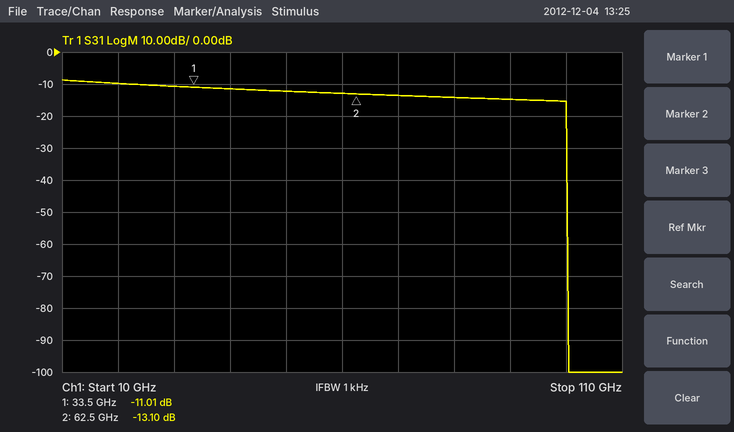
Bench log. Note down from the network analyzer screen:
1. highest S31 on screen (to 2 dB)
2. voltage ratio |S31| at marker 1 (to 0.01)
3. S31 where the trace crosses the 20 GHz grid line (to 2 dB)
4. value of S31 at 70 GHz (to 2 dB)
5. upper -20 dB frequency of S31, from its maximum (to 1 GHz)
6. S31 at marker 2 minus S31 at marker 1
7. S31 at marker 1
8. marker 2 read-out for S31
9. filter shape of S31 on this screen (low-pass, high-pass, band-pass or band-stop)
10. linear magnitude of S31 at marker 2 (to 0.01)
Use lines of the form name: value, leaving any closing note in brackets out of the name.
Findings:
highest S31 on screen: -8 dB
voltage ratio |S31| at marker 1: 0.28
S31 where the trace crosses the 20 GHz grid line: -10 dB
value of S31 at 70 GHz: -14 dB
upper -20 dB frequency of S31, from its maximum: 100 GHz
S31 at marker 2 minus S31 at marker 1: -2.09 dB
S31 at marker 1: -11.01 dB
marker 2 read-out for S31: -13.10 dB
filter shape of S31 on this screen: low-pass
linear magnitude of S31 at marker 2: 0.22
